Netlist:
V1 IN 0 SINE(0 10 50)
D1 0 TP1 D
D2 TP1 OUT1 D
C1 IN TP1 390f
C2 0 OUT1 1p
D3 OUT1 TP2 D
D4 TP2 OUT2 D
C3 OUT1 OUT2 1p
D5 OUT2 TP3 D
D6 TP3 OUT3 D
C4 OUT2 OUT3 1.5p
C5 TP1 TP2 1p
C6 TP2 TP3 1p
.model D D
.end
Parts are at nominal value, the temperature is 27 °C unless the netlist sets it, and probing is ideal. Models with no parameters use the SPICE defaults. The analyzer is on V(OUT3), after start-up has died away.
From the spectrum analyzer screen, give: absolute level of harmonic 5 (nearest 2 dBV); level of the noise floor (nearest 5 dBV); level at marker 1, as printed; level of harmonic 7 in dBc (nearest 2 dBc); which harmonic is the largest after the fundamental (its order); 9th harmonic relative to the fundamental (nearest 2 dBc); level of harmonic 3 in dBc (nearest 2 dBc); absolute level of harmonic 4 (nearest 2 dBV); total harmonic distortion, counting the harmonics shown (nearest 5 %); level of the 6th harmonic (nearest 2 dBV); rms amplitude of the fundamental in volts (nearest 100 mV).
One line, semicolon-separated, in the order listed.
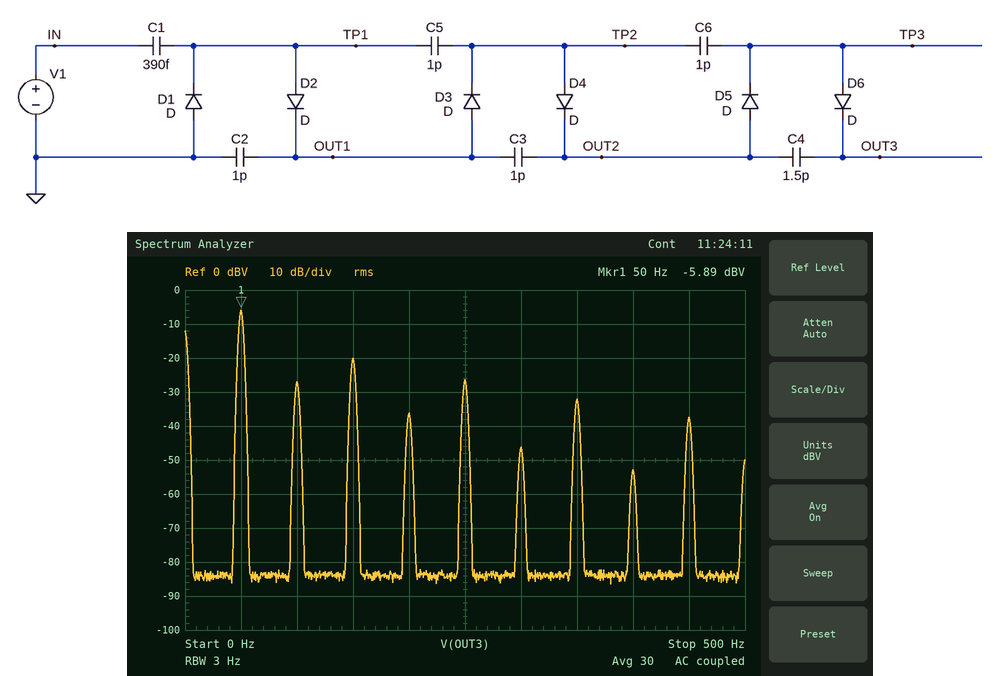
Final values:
-26 dBV; -85 dBV; -5.89 dBV; -26 dBc; 3; -32 dBc; -14 dBc; -36 dBV; 25 %; -46 dBV; 500 mV
